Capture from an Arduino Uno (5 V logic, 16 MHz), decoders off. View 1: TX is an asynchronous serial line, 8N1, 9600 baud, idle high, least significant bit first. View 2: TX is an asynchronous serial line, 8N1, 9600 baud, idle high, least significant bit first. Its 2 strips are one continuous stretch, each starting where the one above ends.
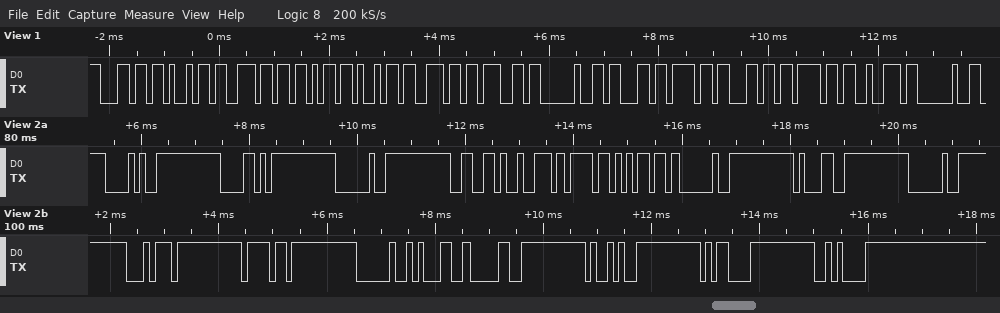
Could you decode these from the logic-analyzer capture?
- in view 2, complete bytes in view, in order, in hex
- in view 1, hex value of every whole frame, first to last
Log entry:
28 58 20 66 72 6F 6D 20 31 20 74 6F 20 31 30 29 0D 0A
6C 69 6E 6B 69 6E 67 20 63 6F 6C 6F 72 20
